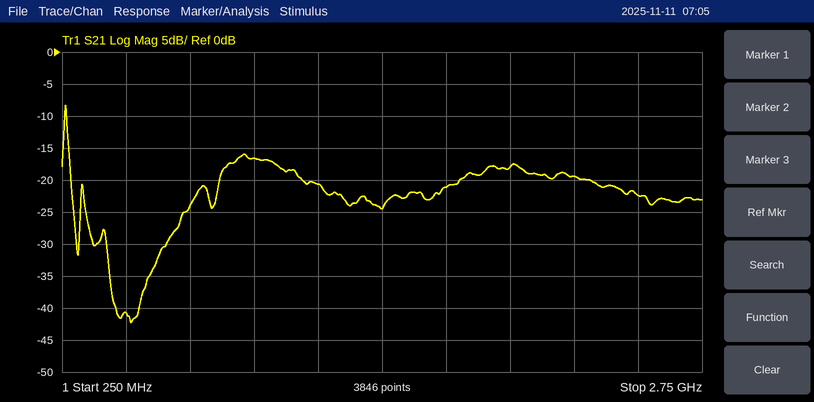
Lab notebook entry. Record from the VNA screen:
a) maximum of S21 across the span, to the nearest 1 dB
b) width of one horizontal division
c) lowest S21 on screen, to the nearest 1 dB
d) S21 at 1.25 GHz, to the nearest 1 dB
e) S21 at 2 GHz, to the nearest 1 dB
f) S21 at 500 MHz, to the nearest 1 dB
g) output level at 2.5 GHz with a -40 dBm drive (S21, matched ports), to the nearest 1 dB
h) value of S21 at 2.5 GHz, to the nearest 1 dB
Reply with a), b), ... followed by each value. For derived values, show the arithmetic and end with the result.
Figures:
a) -8 dB
b) 250 MHz
c) -42 dB
d) -21 dB
e) -18 dB
f) -41 dB
g) -40 dBm + (-22 dB) = -62 dBm
h) -22 dB
